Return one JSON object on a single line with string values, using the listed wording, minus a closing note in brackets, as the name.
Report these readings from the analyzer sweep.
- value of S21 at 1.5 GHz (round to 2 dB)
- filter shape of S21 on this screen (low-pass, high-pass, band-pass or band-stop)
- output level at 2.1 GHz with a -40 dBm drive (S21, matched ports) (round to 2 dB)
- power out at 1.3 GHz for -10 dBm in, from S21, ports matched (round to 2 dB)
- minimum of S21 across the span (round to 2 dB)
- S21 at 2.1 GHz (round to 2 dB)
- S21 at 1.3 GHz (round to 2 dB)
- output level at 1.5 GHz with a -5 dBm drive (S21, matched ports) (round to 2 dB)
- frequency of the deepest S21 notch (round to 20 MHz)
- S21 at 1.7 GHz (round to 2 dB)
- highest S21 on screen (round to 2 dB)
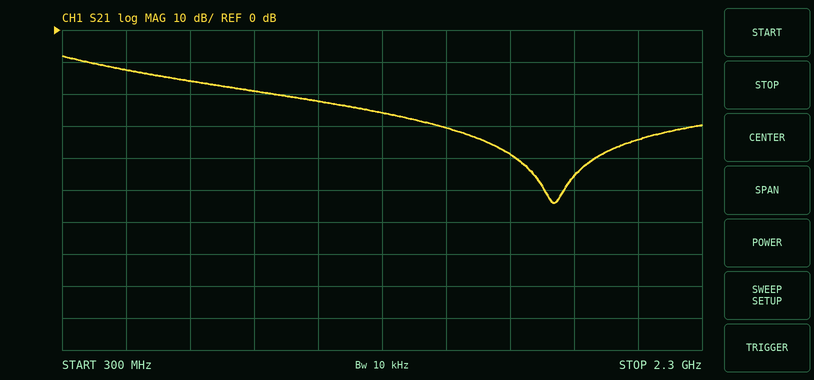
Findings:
{"value of S21 at 1.5 GHz": "-30 dB", "filter shape of S21 on this screen": "low-pass", "output level at 2.1 GHz with a -40 dBm drive (S21, matched ports)": "-74 dBm", "power out at 1.3 GHz for -10 dBm in, from S21, ports matched": "-36 dBm", "minimum of S21 across the span": "-54 dB", "S21 at 2.1 GHz": "-34 dB", "S21 at 1.3 GHz": "-26 dB", "output level at 1.5 GHz with a -5 dBm drive (S21, matched ports)": "-36 dBm", "frequency of the deepest S21 notch": "1.84 GHz", "S21 at 1.7 GHz": "-38 dB", "highest S21 on screen": "-8 dB"}
